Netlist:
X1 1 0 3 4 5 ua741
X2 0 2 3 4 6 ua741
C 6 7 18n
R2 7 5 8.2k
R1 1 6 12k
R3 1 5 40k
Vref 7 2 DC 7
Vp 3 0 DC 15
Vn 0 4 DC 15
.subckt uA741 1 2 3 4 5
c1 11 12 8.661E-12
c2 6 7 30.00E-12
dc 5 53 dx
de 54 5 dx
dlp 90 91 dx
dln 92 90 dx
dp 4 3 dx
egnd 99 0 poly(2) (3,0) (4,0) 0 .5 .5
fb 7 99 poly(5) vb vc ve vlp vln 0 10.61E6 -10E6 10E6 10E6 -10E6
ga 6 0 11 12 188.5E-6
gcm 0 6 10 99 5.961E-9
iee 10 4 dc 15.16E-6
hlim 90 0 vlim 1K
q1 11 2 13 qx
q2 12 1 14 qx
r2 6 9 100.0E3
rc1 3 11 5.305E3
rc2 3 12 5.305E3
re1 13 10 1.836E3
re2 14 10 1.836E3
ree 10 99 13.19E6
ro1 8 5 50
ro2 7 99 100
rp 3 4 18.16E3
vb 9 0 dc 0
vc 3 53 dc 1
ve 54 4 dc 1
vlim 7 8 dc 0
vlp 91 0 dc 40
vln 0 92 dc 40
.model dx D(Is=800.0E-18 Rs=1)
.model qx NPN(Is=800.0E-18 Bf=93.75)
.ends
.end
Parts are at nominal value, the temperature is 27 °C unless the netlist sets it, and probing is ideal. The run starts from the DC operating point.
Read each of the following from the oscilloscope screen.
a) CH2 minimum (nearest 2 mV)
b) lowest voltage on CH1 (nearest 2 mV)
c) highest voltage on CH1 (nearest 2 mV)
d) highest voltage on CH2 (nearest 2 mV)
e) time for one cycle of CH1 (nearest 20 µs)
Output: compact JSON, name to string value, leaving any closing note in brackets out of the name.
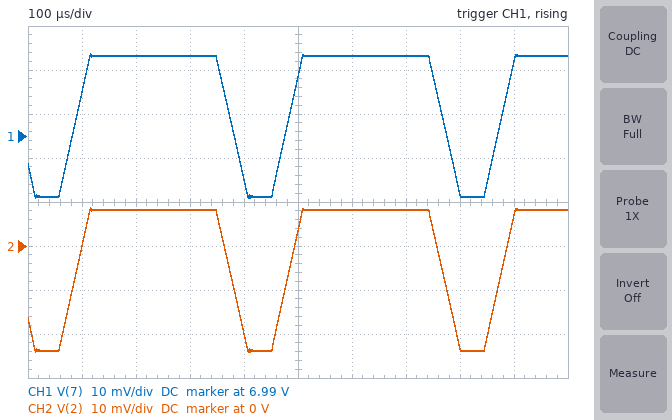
{"CH2 minimum": "-24 mV", "lowest voltage on CH1": "6.976 V", "highest voltage on CH1": "7.008 V", "highest voltage on CH2": "8 mV", "time for one cycle of CH1": "400 µs"}
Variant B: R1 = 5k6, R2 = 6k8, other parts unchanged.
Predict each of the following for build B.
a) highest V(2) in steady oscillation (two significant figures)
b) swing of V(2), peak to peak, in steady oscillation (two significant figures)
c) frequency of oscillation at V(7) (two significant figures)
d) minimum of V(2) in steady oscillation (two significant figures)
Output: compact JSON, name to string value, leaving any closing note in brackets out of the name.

{"highest V(2) in steady oscillation": "10 mV", "swing of V(2), peak to peak, in steady oscillation": "40 mV", "frequency of oscillation at V(7)": "4.0 kHz", "minimum of V(2) in steady oscillation": "-29 mV"}
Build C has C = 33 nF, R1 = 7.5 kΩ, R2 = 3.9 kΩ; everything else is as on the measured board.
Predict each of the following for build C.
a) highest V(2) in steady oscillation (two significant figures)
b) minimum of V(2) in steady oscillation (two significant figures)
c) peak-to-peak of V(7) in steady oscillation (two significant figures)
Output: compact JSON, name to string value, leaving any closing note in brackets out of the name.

{"highest V(2) in steady oscillation": "10 mV", "minimum of V(2) in steady oscillation": "-28 mV", "peak-to-peak of V(7) in steady oscillation": "39 mV"}
